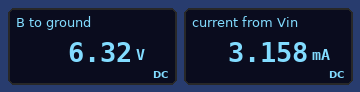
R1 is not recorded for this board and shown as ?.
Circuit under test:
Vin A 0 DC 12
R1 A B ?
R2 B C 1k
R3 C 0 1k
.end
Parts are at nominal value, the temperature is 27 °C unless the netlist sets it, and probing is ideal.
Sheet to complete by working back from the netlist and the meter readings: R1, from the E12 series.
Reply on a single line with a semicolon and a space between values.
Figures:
1.8 kΩ
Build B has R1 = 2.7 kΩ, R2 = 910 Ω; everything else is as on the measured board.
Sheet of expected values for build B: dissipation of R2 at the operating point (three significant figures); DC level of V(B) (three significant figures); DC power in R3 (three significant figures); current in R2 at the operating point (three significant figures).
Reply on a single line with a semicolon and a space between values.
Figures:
6.17 mW; 4.97 V; 6.78 mW; 2.60 mA
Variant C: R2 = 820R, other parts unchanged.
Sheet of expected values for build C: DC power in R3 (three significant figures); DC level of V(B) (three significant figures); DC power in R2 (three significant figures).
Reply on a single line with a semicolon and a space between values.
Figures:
11.0 mW; 6.03 V; 9.01 mW
